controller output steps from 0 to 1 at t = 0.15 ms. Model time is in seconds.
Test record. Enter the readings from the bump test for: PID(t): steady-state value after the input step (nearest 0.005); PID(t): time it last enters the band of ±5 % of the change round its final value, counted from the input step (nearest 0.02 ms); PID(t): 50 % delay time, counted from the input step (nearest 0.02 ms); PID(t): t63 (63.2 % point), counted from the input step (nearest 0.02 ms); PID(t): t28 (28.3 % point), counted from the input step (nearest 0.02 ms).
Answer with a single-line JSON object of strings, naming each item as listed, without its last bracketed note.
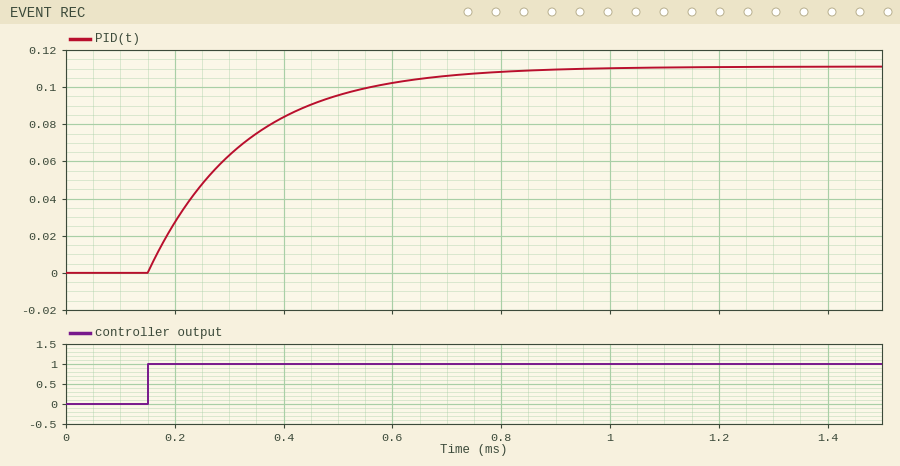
{"PID(t): steady-state value after the input step": "0.110", "PID(t): time it last enters the band of ±5 % of the change round its final value, counted from the input step": "0.54 ms", "PID(t): 50 % delay time, counted from the input step": "0.12 ms", "PID(t): t63 (63.2 % point), counted from the input step": "0.18 ms", "PID(t): t28 (28.3 % point), counted from the input step": "0.06 ms"}
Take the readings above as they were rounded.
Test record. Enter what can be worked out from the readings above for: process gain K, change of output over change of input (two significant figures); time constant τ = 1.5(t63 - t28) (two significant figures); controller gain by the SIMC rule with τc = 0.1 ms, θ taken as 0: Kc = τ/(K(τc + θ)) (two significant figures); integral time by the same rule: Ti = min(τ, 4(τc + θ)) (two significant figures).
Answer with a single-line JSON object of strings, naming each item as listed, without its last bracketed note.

{"process gain K, change of output over change of input": "0.11", "time constant τ = 1.5(t63 - t28)": "0.18 ms", "controller gain by the SIMC rule with τc = 0.1 ms, θ taken as 0: Kc = τ/(K(τc + θ))": "16", "integral time by the same rule: Ti = min(τ, 4(τc + θ))": "0.18 ms"}
